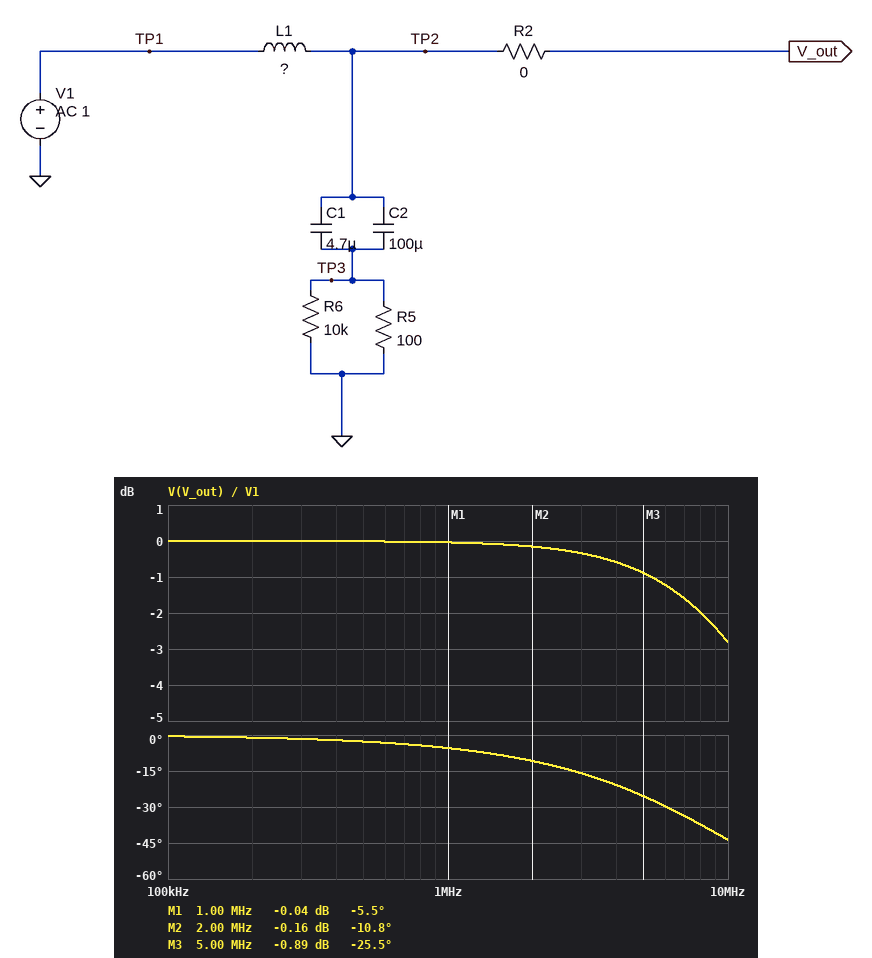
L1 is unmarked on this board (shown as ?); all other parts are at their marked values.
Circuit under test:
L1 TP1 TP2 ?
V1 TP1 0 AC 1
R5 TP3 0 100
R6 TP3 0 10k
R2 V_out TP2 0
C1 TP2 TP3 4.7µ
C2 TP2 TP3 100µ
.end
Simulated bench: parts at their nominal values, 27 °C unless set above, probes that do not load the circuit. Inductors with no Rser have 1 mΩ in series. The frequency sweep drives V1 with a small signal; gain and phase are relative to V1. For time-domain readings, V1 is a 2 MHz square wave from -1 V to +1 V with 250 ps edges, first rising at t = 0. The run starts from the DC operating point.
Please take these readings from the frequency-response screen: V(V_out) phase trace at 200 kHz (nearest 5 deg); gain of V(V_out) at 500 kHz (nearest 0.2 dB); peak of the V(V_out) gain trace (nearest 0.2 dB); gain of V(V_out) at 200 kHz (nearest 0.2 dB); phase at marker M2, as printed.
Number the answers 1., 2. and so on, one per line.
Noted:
1. 0 deg
2. 0 dB
3. 0 dB
4. 0 dB
5. -10.8 deg
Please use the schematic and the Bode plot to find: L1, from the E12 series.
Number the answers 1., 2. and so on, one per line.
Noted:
1. 1.5 µH
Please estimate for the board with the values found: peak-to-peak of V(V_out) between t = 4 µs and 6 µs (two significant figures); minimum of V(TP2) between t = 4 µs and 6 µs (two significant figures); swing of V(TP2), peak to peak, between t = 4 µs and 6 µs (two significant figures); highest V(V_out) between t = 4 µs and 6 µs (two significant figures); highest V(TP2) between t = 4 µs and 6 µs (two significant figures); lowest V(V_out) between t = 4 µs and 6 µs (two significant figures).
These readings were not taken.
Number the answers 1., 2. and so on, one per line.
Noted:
1. 2.0 V
2. -1.0 V
3. 2.0 V
4. 1.0 V
5. 1.0 V
6. -1.0 V
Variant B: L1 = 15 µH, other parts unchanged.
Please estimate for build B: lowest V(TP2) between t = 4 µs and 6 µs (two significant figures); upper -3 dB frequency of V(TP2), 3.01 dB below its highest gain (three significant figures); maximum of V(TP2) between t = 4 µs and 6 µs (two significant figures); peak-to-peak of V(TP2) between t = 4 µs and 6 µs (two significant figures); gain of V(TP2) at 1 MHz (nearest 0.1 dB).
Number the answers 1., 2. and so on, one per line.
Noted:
1. -680 mV
2. 1.05 MHz
3. 680 mV
4. 1.4 V
5. -2.8 dB
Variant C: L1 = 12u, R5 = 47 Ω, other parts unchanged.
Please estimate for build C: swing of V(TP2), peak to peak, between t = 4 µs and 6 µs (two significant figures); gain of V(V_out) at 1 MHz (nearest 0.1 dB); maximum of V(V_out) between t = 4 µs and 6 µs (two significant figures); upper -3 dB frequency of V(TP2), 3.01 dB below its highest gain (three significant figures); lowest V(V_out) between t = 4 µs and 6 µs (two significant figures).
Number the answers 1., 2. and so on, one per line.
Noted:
1. 900 mV
2. -5.6 dB
3. 450 mV
4. 621 kHz
5. -450 mV
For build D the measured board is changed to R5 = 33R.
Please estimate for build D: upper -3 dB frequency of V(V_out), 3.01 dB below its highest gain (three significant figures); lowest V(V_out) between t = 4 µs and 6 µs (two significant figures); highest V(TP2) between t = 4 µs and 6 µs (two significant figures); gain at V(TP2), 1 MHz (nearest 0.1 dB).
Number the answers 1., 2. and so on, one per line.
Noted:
1. 3.49 MHz
2. -990 mV
3. 990 mV
4. -0.3 dB
